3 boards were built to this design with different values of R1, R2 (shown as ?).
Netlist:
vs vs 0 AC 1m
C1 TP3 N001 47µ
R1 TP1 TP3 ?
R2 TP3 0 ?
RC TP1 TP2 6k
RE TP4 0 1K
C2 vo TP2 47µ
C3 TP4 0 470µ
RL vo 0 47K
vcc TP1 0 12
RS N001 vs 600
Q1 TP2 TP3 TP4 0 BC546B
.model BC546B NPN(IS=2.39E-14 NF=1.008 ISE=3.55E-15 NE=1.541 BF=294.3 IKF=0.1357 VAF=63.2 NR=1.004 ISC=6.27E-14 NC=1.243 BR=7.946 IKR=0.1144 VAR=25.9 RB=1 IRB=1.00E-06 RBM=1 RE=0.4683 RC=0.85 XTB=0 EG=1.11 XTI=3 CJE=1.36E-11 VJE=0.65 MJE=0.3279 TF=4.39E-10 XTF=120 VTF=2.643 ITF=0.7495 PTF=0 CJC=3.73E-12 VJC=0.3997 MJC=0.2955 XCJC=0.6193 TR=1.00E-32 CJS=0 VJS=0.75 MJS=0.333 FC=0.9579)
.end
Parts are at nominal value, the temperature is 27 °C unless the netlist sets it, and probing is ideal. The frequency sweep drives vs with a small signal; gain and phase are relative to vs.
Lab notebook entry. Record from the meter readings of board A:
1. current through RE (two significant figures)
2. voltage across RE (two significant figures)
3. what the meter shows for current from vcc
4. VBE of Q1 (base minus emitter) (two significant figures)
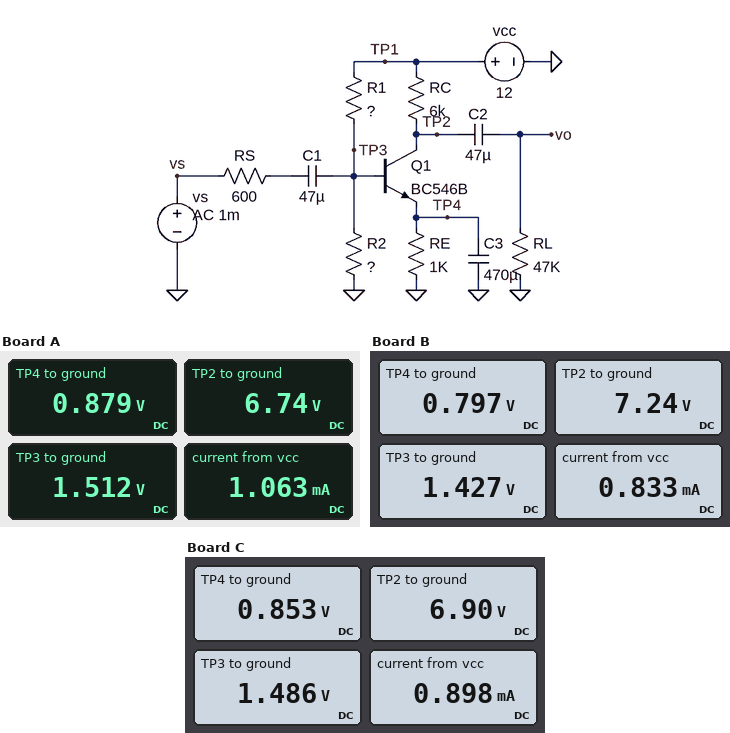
880 µA
880 mV
1.063 mA
630 mV
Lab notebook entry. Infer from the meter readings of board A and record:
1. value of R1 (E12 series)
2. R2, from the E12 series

56 kΩ
8.2 kΩ
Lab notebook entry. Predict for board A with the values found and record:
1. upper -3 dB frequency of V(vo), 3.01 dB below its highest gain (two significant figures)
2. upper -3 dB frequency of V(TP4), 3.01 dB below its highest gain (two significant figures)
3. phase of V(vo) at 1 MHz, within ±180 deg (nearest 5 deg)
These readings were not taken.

870 kHz
11 Hz
130 deg
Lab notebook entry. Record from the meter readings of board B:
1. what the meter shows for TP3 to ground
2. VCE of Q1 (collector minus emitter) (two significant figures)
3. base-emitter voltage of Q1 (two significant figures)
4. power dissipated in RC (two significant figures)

1.427 V
6.4 V
630 mV
3.8 mW
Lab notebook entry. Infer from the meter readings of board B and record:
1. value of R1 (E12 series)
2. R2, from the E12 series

270 kΩ
39 kΩ
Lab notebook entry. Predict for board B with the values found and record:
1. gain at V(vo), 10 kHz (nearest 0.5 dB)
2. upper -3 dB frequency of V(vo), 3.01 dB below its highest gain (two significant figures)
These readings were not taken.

43.0 dB
900 kHz
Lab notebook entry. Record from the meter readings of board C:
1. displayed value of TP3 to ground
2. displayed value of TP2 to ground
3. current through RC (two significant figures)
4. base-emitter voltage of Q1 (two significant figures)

1.486 V
6.90 V
850 µA
630 mV
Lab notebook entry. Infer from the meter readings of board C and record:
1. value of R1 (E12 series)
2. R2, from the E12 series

220 kΩ
33 kΩ
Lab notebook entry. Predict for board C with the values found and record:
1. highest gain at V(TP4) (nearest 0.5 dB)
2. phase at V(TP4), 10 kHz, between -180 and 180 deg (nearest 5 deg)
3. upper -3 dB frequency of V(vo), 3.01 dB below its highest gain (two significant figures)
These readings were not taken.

-1.0 dB
-90 deg
850 kHz
